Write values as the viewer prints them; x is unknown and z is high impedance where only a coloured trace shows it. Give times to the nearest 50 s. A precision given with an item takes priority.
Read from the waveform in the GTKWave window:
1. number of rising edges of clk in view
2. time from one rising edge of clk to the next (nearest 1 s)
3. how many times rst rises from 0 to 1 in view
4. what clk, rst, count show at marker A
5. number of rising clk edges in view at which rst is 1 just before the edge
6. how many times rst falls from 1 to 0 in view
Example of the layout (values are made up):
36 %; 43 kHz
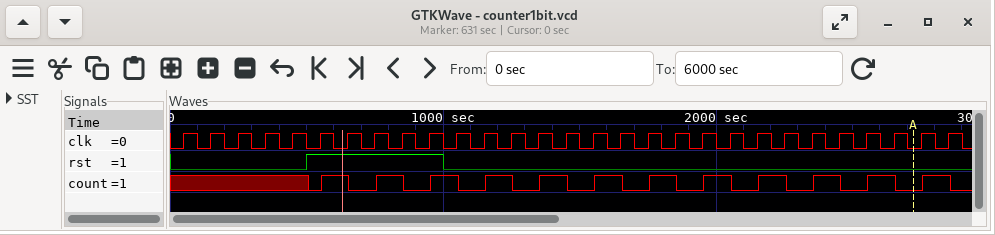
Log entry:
29; 100 s; 1; clk=0, rst=0, count=0; 5; 1
